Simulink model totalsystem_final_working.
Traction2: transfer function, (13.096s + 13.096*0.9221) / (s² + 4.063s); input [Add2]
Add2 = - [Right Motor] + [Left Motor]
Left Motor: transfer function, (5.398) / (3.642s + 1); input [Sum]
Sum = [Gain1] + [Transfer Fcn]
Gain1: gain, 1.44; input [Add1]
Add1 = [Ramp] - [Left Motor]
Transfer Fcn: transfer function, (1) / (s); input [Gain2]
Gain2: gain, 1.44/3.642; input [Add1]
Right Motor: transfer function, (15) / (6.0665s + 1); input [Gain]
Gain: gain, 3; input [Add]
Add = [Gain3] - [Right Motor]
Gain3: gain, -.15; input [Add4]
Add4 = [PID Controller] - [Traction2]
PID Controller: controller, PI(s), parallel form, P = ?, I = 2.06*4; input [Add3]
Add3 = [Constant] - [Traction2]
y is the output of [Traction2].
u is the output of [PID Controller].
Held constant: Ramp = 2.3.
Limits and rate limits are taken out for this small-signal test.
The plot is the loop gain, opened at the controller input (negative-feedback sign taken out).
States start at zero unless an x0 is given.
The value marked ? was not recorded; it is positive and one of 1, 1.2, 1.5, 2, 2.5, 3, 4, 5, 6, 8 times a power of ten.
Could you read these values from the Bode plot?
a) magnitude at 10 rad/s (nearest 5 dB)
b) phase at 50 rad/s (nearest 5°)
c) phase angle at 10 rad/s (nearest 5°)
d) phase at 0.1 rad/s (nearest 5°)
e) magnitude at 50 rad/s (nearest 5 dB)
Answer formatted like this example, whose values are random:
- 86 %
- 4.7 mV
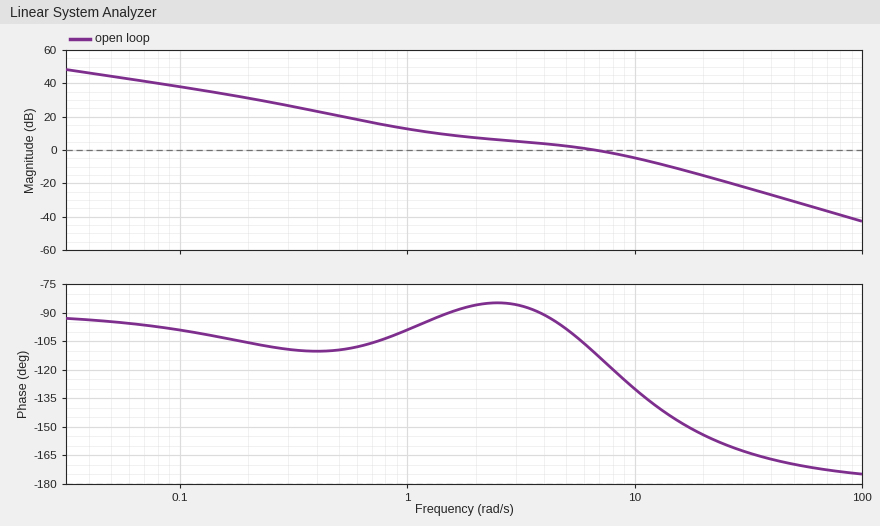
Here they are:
- -5 dB
- -170°
- -130°
- -100°
- -30 dB
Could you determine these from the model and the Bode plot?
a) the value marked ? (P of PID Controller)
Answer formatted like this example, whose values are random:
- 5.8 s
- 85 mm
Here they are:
- 5
